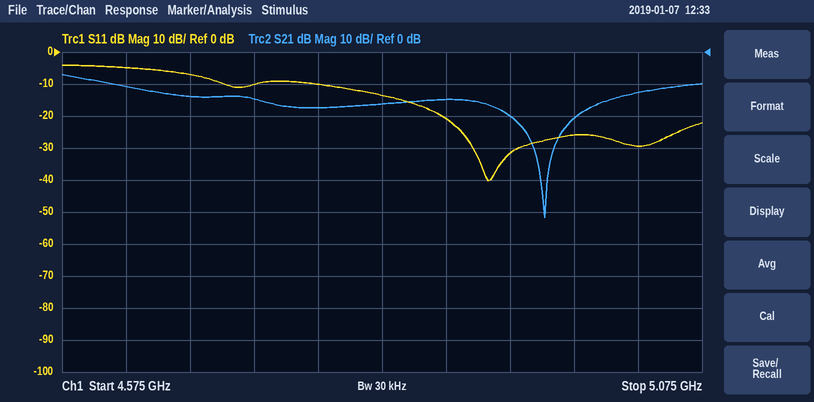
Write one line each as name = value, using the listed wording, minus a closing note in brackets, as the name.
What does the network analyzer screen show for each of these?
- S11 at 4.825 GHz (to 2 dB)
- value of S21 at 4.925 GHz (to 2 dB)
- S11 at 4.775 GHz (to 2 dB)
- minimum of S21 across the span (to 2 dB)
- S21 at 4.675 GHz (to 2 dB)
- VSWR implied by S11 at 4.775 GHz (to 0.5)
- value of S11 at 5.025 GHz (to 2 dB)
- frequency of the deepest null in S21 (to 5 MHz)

S11 at 4.825 GHz = -14 dB
value of S21 at 4.925 GHz = -20 dB
S11 at 4.775 GHz = -10 dB
minimum of S21 across the span = -52 dB
S21 at 4.675 GHz = -14 dB
VSWR implied by S11 at 4.775 GHz = 2.0
value of S11 at 5.025 GHz = -30 dB
frequency of the deepest null in S21 = 4.950 GHz
